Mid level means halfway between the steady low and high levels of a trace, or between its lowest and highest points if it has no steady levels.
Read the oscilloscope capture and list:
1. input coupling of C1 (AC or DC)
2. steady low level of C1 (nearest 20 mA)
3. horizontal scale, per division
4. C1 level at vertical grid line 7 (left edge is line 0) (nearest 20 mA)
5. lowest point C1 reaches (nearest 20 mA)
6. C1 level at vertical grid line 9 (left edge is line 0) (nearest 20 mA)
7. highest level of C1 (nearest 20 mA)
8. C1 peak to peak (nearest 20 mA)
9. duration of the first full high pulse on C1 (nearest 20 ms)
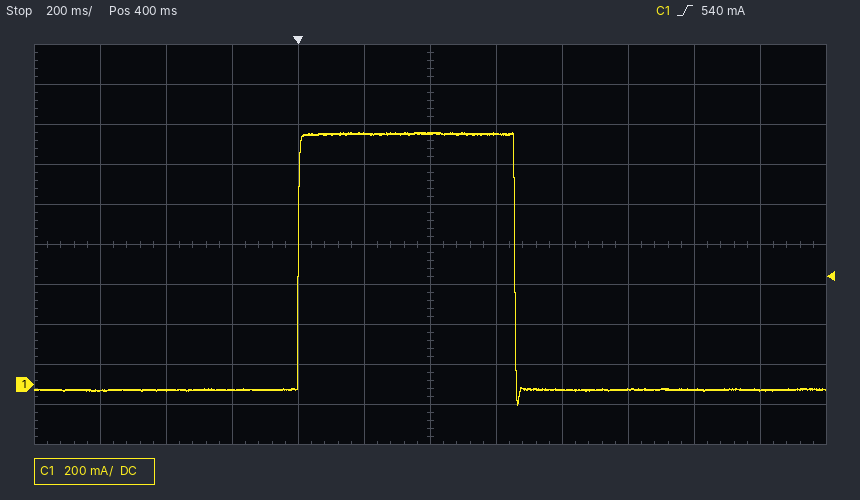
DC
-20 mA
200 ms
1.26 A
-100 mA
-20 mA
1.26 A
1.36 A
660 ms
